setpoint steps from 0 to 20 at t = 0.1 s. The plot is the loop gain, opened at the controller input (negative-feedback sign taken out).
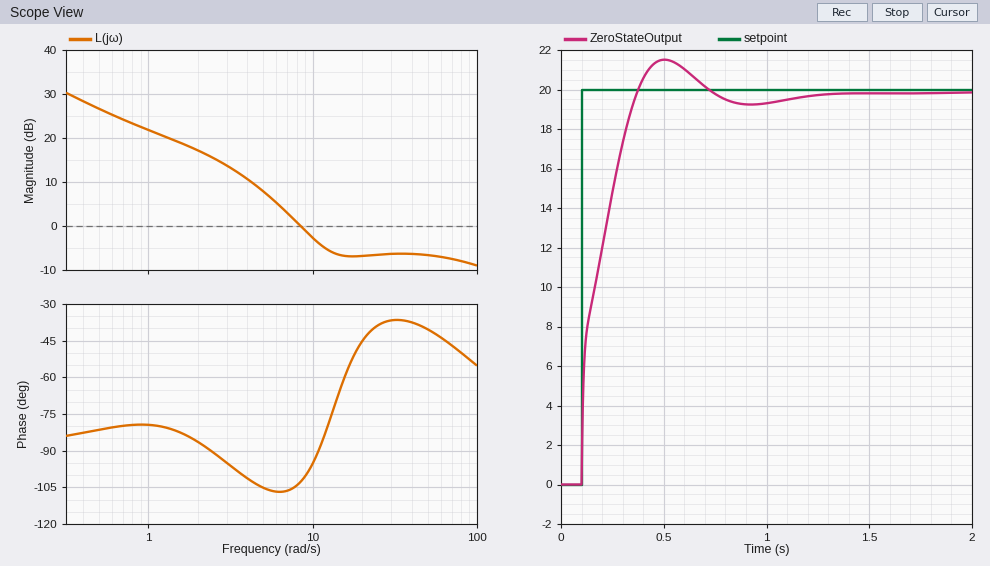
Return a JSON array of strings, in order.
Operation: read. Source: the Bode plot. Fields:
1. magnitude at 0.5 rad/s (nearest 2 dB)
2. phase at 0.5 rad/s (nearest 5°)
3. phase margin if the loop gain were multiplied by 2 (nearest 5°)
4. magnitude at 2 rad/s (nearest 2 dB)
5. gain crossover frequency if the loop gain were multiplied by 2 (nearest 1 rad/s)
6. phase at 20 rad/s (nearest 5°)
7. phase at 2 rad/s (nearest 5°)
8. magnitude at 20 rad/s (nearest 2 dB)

["26 dB", "-80°", "105°", "18 dB", "13 rad/s", "-45°", "-85°", "-6 dB"]
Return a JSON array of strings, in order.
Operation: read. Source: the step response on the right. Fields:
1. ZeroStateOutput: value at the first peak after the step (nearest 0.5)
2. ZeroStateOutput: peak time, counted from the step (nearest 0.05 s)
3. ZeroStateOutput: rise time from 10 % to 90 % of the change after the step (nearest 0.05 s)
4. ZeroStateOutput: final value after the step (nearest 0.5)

["21.5", "0.40 s", "0.20 s", "20.0"]
